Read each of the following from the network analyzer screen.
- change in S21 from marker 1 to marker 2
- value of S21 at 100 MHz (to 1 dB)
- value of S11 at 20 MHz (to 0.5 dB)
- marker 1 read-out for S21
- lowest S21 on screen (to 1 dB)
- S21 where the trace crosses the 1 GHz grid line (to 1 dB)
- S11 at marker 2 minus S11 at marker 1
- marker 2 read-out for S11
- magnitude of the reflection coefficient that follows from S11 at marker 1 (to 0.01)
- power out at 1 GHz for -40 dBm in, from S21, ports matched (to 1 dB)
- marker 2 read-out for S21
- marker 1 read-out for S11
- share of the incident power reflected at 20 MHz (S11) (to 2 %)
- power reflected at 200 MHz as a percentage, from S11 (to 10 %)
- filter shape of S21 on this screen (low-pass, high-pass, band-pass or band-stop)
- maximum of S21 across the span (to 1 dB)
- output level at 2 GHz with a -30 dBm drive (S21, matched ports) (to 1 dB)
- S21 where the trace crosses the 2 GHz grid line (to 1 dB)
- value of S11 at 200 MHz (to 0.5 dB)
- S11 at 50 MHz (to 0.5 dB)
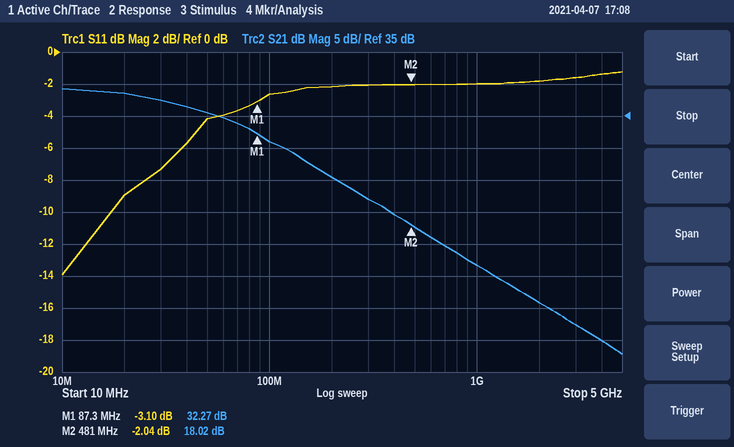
-14.25 dB
31 dB
-9.0 dB
32.27 dB
-2 dB
12 dB
1.06 dB
-2.04 dB
0.70
-28 dBm
18.02 dB
-3.10 dB
12 %
60 %
low-pass
39 dB
-24 dBm
6 dB
-2.0 dB
-4.0 dB
